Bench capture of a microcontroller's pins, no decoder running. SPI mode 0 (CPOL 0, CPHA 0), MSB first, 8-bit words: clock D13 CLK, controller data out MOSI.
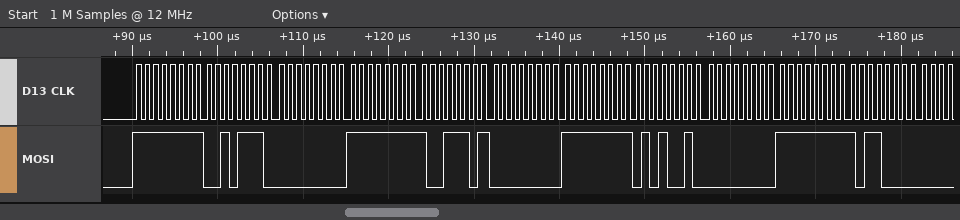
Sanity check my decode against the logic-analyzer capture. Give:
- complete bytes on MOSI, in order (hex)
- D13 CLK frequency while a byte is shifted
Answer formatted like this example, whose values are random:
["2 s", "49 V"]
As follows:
["FF 2E 00 FF 9D 00 FF 52 00 FF B0", "1 MHz"]
